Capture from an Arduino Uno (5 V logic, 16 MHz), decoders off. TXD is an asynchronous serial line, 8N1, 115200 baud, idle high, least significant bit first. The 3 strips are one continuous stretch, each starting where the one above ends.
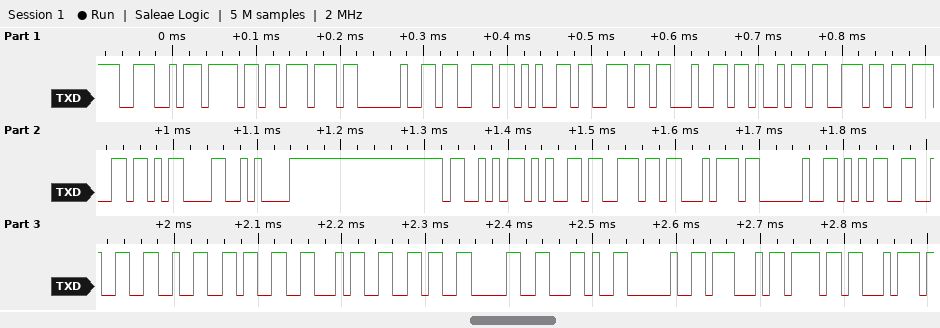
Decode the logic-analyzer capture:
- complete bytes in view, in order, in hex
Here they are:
4E 6F 77 20 73 65 6E 64 69 6E 67 0D 0A 53 65 6E 74 20 35 32 32 33 34 36 30 2C 20 47 6F 74
